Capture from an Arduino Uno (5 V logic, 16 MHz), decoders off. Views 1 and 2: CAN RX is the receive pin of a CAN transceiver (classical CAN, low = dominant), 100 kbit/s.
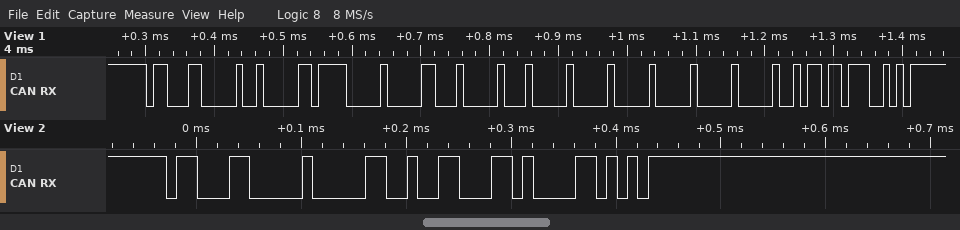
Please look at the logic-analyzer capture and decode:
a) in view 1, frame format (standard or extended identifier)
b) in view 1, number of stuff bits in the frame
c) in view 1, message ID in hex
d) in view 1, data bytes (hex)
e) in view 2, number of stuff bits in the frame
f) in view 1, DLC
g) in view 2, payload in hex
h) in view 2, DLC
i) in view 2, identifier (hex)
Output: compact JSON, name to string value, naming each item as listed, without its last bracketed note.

{"in view 1, frame format": "standard", "in view 1, number of stuff bits in the frame": "11", "in view 1, message ID in hex": "0x630", "in view 1, data bytes": "2F 00 22 01 00 00 00 00", "in view 2, number of stuff bits in the frame": "2", "in view 1, DLC": "8", "in view 2, payload in hex": "26", "in view 2, DLC": "1", "in view 2, identifier": "0x630"}
